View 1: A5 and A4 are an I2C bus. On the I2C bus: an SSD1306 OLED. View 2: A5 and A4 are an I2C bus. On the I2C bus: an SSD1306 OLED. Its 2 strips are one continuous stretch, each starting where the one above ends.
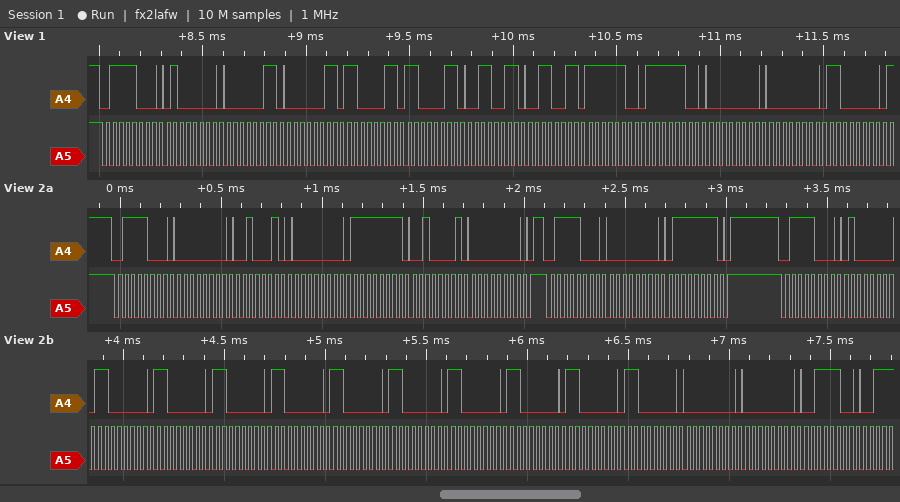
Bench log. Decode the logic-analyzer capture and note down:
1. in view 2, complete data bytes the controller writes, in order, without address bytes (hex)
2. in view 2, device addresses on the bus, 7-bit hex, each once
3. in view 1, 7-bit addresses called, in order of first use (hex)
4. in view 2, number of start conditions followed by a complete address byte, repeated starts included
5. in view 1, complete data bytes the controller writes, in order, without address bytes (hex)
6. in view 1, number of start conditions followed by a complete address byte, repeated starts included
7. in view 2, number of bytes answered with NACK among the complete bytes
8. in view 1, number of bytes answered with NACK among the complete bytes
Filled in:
00 22 00 FF 21 00 00 7F 40 C0 C0 C0 C0 C0 C0 C0 C0 C0 C0 00 00 3C
0x3C
0x3C
3
40 03 03 C3 C3 33 33 FC FC 00 00 C0
1
0
0
